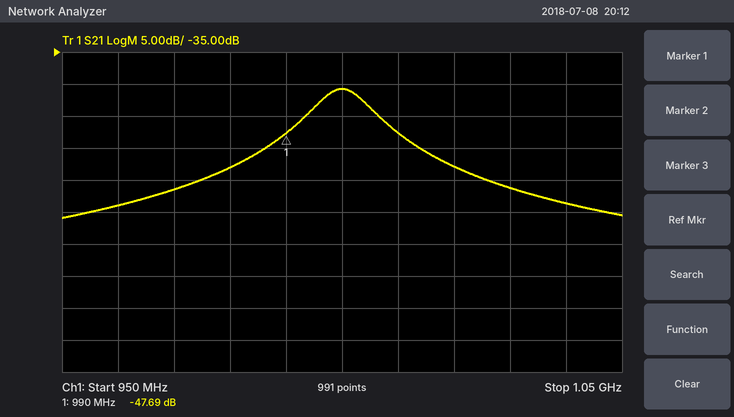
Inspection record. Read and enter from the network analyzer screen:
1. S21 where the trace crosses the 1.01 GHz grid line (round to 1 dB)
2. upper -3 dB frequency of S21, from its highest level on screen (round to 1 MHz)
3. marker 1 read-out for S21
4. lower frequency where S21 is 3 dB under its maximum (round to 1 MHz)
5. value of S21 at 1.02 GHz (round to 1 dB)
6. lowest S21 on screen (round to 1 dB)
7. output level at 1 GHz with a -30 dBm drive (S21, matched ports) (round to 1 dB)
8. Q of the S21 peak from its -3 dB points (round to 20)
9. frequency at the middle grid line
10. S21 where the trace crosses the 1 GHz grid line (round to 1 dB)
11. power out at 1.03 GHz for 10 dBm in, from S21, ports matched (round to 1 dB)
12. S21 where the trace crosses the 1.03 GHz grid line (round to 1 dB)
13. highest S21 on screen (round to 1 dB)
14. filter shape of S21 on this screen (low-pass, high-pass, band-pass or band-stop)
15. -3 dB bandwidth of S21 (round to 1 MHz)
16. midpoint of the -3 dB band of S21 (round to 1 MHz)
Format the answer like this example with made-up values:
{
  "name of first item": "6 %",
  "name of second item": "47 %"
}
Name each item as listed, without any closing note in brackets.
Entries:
{
  "S21 where the trace crosses the 1.01 GHz grid line": "-48 dB",
  "upper -3 dB frequency of S21, from its highest level on screen": "1.005 GHz",
  "marker 1 read-out for S21": "-47.69 dB",
  "lower frequency where S21 is 3 dB under its maximum": "995 MHz",
  "value of S21 at 1.02 GHz": "-53 dB",
  "lowest S21 on screen": "-61 dB",
  "output level at 1 GHz with a -30 dBm drive (S21, matched ports)": "-71 dBm",
  "Q of the S21 peak from its -3 dB points": "100",
  "frequency at the middle grid line": "1 GHz",
  "S21 where the trace crosses the 1 GHz grid line": "-41 dB",
  "power out at 1.03 GHz for 10 dBm in, from S21, ports matched": "-46 dBm",
  "S21 where the trace crosses the 1.03 GHz grid line": "-56 dB",
  "highest S21 on screen": "-41 dB",
  "filter shape of S21 on this screen": "band-pass",
  "-3 dB bandwidth of S21": "10 MHz",
  "midpoint of the -3 dB band of S21": "1.000 GHz"
}
